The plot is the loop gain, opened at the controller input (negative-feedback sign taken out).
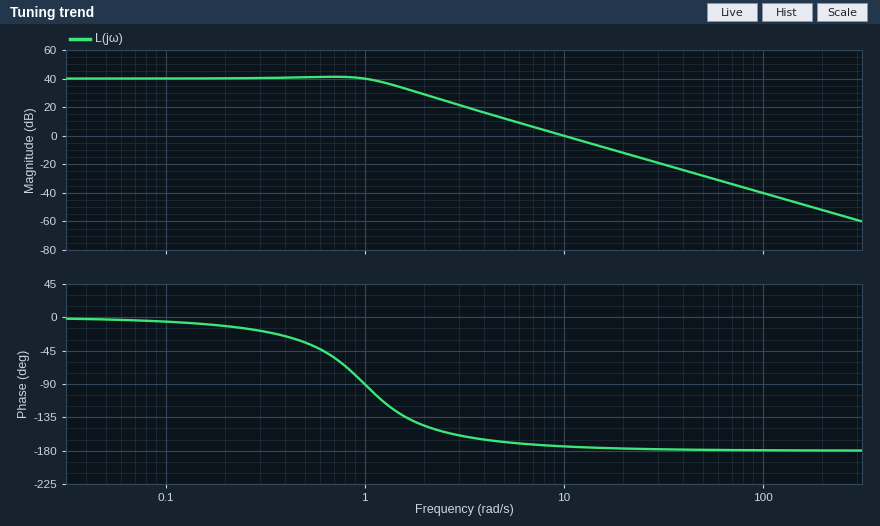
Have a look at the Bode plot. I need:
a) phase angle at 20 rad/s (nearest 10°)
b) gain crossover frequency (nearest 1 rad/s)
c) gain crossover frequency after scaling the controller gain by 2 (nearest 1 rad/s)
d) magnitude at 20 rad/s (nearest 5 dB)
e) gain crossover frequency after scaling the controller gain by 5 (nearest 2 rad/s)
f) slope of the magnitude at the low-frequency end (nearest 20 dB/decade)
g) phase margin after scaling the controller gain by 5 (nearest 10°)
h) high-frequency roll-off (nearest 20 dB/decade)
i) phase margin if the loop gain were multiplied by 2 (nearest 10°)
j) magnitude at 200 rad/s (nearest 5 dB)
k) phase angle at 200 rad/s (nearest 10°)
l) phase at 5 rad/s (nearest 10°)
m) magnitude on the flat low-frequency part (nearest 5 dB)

-180°
10 rad/s
14 rad/s
-10 dB
22 rad/s
0 dB/decade
0°
-40 dB/decade
0°
-50 dB
-180°
-170°
40 dB
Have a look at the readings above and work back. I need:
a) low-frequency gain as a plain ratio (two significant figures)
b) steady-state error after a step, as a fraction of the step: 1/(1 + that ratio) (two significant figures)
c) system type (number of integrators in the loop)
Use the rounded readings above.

100
0.0099
0
